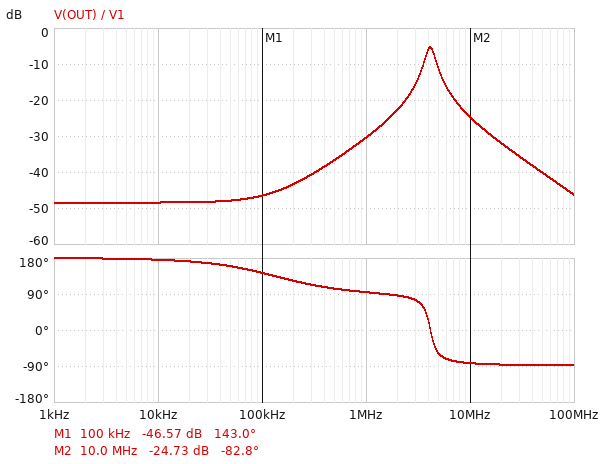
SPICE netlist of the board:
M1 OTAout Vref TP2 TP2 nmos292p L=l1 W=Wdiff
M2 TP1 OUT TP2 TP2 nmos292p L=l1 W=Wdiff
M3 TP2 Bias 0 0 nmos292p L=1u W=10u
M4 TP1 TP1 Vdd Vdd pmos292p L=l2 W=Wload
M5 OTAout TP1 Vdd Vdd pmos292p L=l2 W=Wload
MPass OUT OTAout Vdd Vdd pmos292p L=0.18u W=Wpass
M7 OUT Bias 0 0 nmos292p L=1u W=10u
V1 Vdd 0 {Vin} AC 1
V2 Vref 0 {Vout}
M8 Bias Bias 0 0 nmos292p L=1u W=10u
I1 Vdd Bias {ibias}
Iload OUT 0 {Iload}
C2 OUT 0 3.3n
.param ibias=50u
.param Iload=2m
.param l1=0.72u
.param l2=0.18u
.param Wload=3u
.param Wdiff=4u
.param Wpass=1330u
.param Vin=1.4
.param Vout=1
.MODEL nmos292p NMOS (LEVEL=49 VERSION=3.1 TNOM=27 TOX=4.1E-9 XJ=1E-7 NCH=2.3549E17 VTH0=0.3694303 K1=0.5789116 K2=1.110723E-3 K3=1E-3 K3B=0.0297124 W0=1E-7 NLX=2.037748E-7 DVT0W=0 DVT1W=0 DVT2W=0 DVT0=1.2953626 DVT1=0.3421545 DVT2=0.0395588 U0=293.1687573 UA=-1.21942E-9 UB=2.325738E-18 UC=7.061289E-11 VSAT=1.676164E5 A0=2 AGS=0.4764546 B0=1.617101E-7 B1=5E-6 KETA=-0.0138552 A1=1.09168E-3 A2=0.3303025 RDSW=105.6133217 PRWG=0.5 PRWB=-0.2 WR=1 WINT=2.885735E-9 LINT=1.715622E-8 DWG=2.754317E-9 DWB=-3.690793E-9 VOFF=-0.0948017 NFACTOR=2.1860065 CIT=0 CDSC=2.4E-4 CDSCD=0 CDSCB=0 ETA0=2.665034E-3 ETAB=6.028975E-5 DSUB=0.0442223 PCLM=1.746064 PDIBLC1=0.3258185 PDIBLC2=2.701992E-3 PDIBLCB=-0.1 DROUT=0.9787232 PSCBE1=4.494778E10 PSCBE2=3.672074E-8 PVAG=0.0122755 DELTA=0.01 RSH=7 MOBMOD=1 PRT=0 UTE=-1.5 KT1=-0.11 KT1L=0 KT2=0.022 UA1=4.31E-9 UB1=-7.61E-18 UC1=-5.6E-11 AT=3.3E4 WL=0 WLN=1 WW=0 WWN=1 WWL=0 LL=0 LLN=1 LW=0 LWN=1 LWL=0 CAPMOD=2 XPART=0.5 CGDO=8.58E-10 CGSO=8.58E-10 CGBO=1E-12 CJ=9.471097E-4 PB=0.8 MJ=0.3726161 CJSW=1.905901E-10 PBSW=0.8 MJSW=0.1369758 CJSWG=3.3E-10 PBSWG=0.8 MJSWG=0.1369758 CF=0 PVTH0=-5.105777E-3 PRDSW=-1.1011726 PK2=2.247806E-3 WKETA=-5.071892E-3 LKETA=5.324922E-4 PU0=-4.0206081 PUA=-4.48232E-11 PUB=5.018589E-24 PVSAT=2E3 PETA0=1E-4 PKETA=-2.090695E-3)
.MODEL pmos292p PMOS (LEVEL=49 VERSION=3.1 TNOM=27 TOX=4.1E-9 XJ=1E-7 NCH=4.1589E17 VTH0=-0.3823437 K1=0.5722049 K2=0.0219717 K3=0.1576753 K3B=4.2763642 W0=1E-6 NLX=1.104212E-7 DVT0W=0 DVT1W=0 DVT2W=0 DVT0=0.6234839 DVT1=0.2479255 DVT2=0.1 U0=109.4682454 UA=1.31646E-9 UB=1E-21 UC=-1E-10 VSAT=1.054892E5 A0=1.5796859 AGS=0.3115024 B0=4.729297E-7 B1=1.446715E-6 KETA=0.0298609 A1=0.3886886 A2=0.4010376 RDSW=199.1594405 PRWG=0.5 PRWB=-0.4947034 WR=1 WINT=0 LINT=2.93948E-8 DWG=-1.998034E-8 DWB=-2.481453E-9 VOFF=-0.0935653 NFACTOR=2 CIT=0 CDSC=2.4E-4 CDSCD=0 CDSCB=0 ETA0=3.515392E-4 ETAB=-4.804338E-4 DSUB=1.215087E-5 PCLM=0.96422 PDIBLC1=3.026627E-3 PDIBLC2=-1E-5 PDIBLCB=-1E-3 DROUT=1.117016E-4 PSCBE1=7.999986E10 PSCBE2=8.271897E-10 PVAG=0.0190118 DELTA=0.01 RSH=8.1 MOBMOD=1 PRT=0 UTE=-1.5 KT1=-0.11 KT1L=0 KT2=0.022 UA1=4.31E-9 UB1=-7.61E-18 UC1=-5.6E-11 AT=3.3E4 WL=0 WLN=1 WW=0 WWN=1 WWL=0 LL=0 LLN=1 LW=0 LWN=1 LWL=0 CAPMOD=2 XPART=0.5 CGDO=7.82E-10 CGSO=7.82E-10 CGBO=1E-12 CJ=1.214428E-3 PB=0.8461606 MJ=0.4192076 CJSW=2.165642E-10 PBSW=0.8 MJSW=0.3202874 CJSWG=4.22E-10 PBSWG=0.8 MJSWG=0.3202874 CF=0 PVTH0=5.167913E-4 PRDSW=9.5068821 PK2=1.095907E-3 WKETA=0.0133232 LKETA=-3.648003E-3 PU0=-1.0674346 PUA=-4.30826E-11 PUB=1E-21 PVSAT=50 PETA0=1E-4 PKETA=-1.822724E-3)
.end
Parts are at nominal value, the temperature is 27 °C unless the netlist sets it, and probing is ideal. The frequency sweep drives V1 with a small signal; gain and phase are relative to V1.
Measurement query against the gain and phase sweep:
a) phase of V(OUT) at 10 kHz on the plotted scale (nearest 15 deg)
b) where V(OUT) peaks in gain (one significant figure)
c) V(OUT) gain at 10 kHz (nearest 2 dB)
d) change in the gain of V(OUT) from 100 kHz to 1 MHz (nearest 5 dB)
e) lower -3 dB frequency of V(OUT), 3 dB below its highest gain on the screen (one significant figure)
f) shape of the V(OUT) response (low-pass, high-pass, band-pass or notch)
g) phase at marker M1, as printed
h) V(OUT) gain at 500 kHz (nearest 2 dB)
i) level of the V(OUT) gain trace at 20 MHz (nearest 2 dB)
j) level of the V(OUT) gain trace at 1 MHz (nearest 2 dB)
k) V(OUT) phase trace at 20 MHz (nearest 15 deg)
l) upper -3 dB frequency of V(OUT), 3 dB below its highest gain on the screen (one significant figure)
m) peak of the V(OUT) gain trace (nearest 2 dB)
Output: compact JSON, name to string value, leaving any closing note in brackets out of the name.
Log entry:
{"phase of V(OUT) at 10 kHz on the plotted scale": "180 deg", "where V(OUT) peaks in gain": "4 MHz", "V(OUT) gain at 10 kHz": "-48 dB", "change in the gain of V(OUT) from 100 kHz to 1 MHz": "15 dB", "lower -3 dB frequency of V(OUT), 3 dB below its highest gain on the screen": "4 MHz", "shape of the V(OUT) response": "band-pass", "phase at marker M1, as printed": "143.0 deg", "V(OUT) gain at 500 kHz": "-36 dB", "level of the V(OUT) gain trace at 20 MHz": "-32 dB", "level of the V(OUT) gain trace at 1 MHz": "-30 dB", "V(OUT) phase trace at 20 MHz": "-90 deg", "upper -3 dB frequency of V(OUT), 3 dB below its highest gain on the screen": "5 MHz", "peak of the V(OUT) gain trace": "-6 dB"}
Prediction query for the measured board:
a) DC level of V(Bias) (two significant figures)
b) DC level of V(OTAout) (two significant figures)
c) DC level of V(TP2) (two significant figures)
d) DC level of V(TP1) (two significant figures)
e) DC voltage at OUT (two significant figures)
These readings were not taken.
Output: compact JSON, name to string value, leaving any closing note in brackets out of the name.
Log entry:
{"DC level of V(Bias)": "620 mV", "DC level of V(OTAout)": "840 mV", "DC level of V(TP2)": "380 mV", "DC level of V(TP1)": "750 mV", "DC voltage at OUT": "1.0 V"}
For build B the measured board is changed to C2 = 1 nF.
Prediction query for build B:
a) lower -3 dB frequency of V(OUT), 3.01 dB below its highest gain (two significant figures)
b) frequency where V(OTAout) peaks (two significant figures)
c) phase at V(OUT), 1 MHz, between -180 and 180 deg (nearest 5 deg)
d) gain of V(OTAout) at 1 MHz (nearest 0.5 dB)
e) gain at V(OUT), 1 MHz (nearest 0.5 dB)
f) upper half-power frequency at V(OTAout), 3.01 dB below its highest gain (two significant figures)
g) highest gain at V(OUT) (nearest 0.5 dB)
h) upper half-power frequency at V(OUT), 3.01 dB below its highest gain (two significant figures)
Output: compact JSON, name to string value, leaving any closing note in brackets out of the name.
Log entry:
{"lower -3 dB frequency of V(OUT), 3.01 dB below its highest gain": "6.6 MHz", "frequency where V(OTAout) peaks": "7.1 MHz", "phase at V(OUT), 1 MHz, between -180 and 180 deg": "95 deg", "gain of V(OTAout) at 1 MHz": "0 dB", "gain at V(OUT), 1 MHz": "-31.0 dB", "upper half-power frequency at V(OTAout), 3.01 dB below its highest gain": "8.0 MHz", "highest gain at V(OUT)": "-2.0 dB", "upper half-power frequency at V(OUT), 3.01 dB below its highest gain": "8.6 MHz"}
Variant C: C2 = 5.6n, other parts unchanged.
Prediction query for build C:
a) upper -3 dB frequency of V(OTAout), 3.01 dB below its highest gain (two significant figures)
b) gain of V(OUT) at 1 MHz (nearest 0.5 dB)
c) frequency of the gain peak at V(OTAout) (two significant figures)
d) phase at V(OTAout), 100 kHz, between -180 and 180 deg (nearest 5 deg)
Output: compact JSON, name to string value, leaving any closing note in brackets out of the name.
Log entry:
{"upper -3 dB frequency of V(OTAout), 3.01 dB below its highest gain": "3.4 MHz", "gain of V(OUT) at 1 MHz": "-30.0 dB", "frequency of the gain peak at V(OTAout)": "3.1 MHz", "phase at V(OTAout), 100 kHz, between -180 and 180 deg": "0 deg"}
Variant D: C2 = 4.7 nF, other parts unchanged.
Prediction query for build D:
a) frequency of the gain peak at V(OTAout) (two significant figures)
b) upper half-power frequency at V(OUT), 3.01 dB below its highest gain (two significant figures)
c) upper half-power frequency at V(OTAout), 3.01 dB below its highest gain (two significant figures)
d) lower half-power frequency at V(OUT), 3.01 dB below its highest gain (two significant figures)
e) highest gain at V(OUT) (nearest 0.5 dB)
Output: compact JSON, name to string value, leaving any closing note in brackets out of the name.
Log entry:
{"frequency of the gain peak at V(OTAout)": "3.3 MHz", "upper half-power frequency at V(OUT), 3.01 dB below its highest gain": "3.9 MHz", "upper half-power frequency at V(OTAout), 3.01 dB below its highest gain": "3.7 MHz", "lower half-power frequency at V(OUT), 3.01 dB below its highest gain": "3.1 MHz", "highest gain at V(OUT)": "-7.0 dB"}
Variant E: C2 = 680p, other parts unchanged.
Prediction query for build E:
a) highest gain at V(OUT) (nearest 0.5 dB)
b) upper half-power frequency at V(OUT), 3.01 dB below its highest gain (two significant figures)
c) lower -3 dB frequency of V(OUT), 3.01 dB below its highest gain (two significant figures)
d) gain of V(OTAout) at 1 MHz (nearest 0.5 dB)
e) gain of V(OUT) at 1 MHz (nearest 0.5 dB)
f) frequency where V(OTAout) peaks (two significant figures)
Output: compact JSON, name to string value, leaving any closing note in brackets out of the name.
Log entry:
{"highest gain at V(OUT)": "-1.0 dB", "upper half-power frequency at V(OUT), 3.01 dB below its highest gain": "11 MHz", "lower -3 dB frequency of V(OUT), 3.01 dB below its highest gain": "7.9 MHz", "gain of V(OTAout) at 1 MHz": "0 dB", "gain of V(OUT) at 1 MHz": "-31.0 dB", "frequency where V(OTAout) peaks": "8.6 MHz"}
